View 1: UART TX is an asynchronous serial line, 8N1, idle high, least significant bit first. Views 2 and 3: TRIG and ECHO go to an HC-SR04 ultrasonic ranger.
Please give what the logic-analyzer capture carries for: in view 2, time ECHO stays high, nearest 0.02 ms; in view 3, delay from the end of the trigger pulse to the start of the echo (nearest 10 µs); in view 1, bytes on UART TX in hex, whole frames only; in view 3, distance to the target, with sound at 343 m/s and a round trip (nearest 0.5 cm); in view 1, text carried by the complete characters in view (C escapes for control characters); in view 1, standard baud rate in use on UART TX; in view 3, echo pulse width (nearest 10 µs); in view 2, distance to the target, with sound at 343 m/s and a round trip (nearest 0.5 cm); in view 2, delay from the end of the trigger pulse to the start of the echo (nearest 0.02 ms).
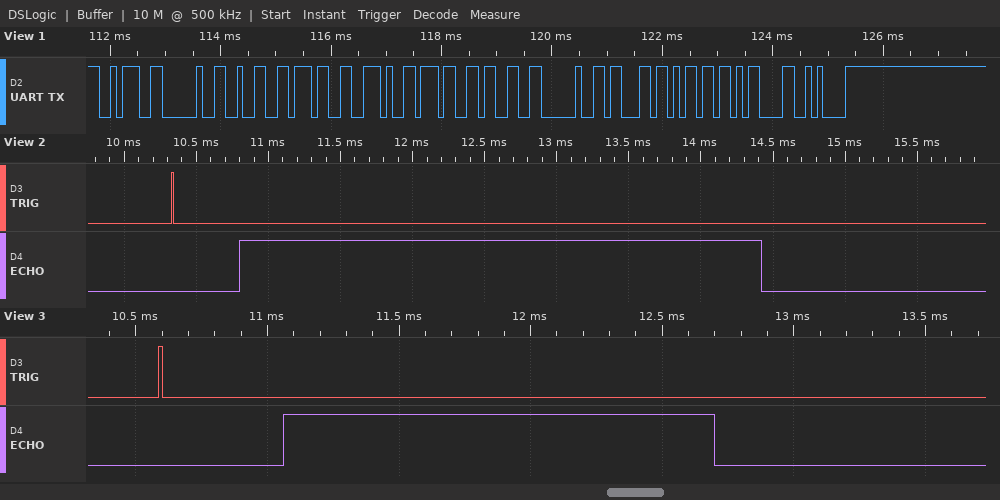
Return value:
3.62 ms
460 µs
0x3A 0x20 0x32 0x37 0x2E 0x37 0x33 0x20 0x63 0x6D 0x0D 0x0A
28 cm
": 27.73 cm\r\n"
9600 baud
1640 µs
62 cm
0.46 ms
